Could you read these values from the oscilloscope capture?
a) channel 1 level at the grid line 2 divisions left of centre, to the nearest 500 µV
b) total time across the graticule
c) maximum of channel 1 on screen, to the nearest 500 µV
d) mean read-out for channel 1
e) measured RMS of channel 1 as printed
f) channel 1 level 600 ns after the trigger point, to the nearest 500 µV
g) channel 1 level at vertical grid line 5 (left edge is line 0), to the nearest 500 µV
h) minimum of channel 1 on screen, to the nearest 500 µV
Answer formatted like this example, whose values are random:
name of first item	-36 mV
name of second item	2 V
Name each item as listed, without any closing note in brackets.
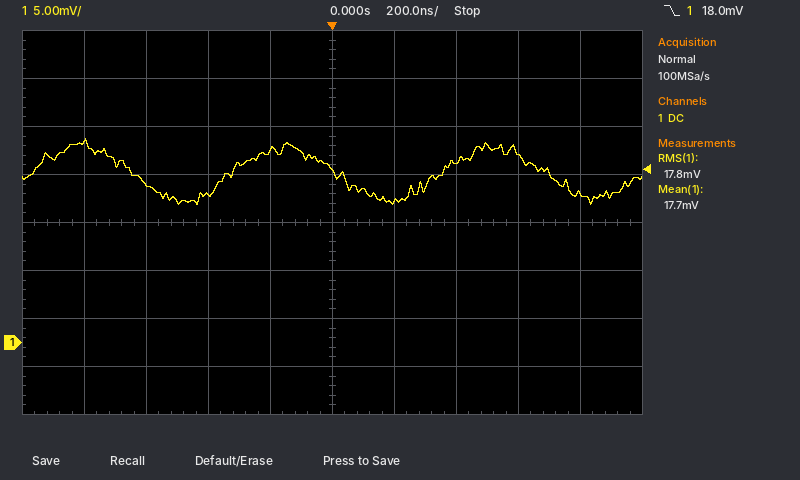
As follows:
channel 1 level at the grid line 2 divisions left of centre, to the nearest 500 µV	15.5 mV
total time across the graticule	2 µs
maximum of channel 1 on screen, to the nearest 500 µV	21.0 mV
mean read-out for channel 1	17.7 mV
measured RMS of channel 1 as printed	17.8 mV
channel 1 level 600 ns after the trigger point, to the nearest 500 µV	19.5 mV
channel 1 level at vertical grid line 5 (left edge is line 0), to the nearest 500 µV	18.0 mV
minimum of channel 1 on screen, to the nearest 500 µV	14.5 mV
